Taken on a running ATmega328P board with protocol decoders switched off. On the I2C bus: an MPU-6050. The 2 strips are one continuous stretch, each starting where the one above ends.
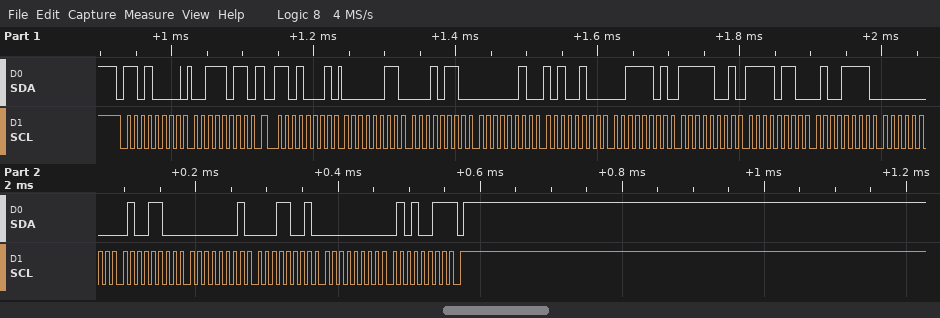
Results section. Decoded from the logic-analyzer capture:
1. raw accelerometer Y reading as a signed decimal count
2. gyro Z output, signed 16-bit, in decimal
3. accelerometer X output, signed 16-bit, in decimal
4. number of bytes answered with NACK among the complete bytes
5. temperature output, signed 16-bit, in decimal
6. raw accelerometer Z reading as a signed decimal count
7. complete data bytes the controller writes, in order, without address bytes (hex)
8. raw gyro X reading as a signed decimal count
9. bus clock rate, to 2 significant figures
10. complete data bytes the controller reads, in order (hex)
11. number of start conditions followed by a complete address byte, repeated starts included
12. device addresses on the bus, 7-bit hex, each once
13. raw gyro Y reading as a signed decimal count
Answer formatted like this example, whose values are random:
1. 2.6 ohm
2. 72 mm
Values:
1. 676
2. 83
3. 790
4. 1
5. -2481
6. 15865
7. 3B
8. 76
9. 100 kHz
10. 03 16 02 A4 3D F9 F6 4F 00 4C 01 19 00 53
11. 2
12. 0x68
13. 281
